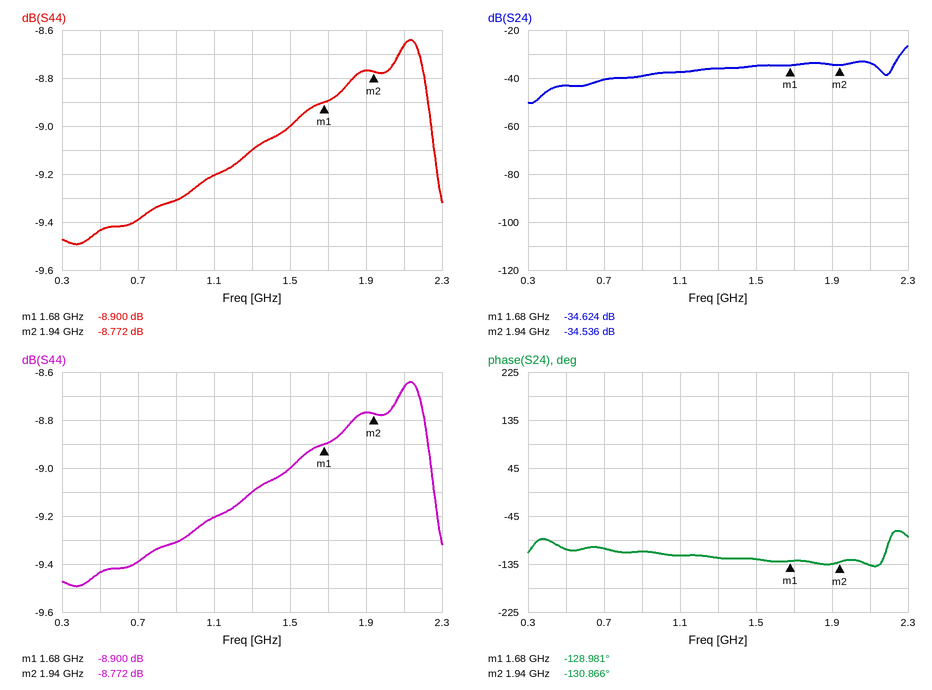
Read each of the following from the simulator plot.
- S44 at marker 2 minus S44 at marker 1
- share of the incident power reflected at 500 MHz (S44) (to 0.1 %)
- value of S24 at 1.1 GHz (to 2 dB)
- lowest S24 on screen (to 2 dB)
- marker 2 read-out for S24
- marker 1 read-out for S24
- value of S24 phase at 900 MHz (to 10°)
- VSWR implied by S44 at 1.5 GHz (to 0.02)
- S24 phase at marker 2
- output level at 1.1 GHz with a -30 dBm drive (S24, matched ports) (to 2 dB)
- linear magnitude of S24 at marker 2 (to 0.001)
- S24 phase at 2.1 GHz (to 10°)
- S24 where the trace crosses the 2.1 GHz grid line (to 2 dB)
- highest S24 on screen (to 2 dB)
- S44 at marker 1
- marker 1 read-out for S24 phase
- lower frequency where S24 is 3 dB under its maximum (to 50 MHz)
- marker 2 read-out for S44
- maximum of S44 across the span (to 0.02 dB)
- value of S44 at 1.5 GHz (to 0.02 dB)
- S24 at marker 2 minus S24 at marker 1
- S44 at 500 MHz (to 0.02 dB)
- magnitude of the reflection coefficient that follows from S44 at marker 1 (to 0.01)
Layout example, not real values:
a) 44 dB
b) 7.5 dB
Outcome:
a) 0.128 dB
b) 11.4 %
c) -38 dB
d) -50 dB
e) -34.536 dB
f) -34.624 dB
g) -110°
h) 2.10
i) -130.866°
j) -68 dBm
k) 0.019
l) -140°
m) -34 dB
n) -26 dB
o) -8.900 dB
p) -128.981°
q) 2.25 GHz
r) -8.772 dB
s) -8.64 dB
t) -9.00 dB
u) 0.088 dB
v) -9.44 dB
w) 0.36
